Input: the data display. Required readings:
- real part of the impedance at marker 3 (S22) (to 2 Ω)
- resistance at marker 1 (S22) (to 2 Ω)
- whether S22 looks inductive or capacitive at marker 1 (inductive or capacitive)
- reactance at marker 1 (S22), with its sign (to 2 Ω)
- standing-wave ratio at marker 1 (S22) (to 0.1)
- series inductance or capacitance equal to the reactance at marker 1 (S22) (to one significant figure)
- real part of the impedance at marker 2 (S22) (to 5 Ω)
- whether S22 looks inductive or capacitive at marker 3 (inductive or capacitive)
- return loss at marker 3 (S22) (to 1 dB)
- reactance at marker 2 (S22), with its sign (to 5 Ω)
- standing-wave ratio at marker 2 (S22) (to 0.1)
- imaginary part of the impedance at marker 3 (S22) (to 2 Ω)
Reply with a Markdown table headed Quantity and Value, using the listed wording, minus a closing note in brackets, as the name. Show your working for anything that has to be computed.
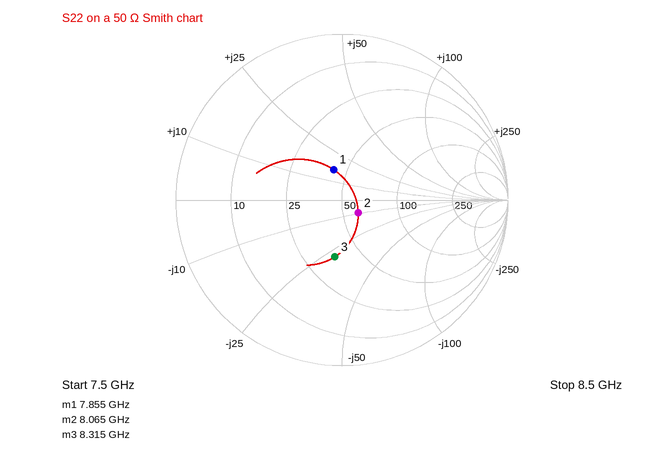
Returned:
| Quantity | Value |
|---|---|
| real part of the impedance at marker 3 (S22) | 36 Ω |
| resistance at marker 1 (S22) | 42 Ω |
| whether S22 looks inductive or capacitive at marker 1 | inductive |
| reactance at marker 1 (S22), with its sign | +16 Ω |
| standing-wave ratio at marker 1 (S22) | 1.5 |
| series inductance or capacitance equal to the reactance at marker 1 (S22) | L = 16 Ω/(2π × 7.855 GHz) ≈ 324 pH, so 300 pH to one significant figure |
| real part of the impedance at marker 2 (S22) | 60 Ω |
| whether S22 looks inductive or capacitive at marker 3 | capacitive |
| return loss at marker 3 (S22) | 9 dB |
| reactance at marker 2 (S22), with its sign | -10 Ω |
| standing-wave ratio at marker 2 (S22) | 1.3 |
| imaginary part of the impedance at marker 3 (S22) | -28 Ω |
